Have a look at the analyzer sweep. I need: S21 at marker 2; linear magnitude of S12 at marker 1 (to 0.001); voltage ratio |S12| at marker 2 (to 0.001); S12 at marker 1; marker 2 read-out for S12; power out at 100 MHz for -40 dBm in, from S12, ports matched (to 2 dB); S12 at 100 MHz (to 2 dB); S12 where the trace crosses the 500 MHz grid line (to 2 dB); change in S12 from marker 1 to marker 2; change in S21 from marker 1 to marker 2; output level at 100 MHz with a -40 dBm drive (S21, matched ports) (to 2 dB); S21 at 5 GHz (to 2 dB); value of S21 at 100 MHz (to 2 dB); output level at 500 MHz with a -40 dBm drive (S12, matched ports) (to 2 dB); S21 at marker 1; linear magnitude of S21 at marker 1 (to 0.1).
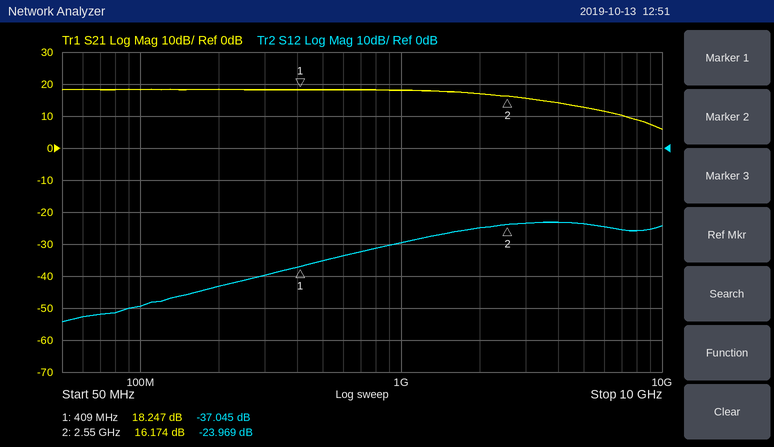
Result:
16.174 dB
0.014
0.063
-37.045 dB
-23.969 dB
-90 dBm
-50 dB
-36 dB
13.076 dB
-2.073 dB
-22 dBm
12 dB
18 dB
-76 dBm
18.247 dB
8.2
